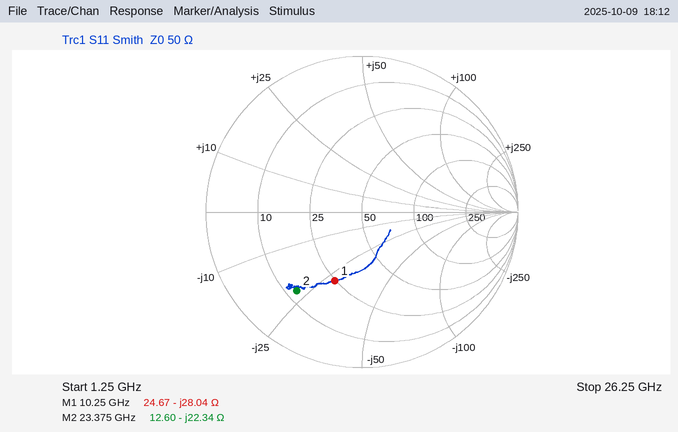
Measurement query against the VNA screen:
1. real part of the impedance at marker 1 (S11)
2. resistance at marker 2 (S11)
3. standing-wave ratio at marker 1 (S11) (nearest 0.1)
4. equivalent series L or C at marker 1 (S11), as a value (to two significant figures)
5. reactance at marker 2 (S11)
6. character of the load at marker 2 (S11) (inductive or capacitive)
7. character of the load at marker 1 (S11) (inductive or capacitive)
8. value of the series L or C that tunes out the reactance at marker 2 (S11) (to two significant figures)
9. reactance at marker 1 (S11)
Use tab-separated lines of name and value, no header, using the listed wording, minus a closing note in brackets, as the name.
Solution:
real part of the impedance at marker 1	24.67 Ω
resistance at marker 2	12.60 Ω
standing-wave ratio at marker 1 (S11)	2.8
equivalent series L or C at marker 1 (S11), as a value	550 fF
reactance at marker 2	-22.34 Ω
character of the load at marker 2 (S11)	capacitive
character of the load at marker 1 (S11)	capacitive
value of the series L or C that tunes out the reactance at marker 2 (S11)	150 pH
reactance at marker 1	-28.04 Ω
